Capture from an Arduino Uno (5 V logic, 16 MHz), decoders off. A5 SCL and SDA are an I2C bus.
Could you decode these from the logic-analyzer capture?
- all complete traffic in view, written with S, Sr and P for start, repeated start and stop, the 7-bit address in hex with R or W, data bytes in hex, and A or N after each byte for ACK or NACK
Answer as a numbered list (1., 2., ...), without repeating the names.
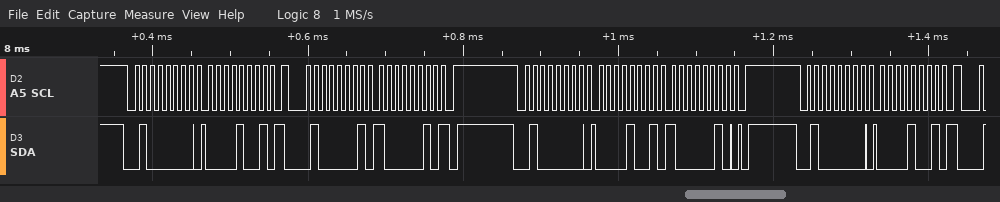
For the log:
1. S 20W A 09 A Sr 20R A 82 N P S 20W A 09 A 82 A P S 20W A 09 A
